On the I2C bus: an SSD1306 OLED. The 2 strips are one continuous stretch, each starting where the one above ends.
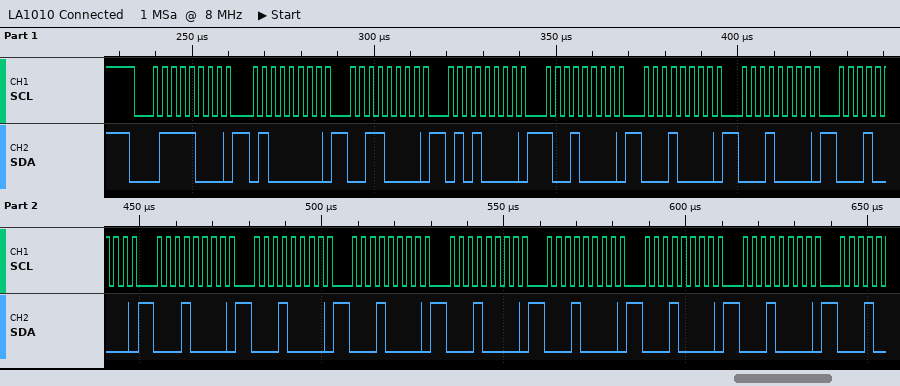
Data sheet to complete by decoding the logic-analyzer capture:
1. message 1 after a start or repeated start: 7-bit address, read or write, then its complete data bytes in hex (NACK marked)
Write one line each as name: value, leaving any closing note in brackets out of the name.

message 1 after a start or repeated start: 7-bit address, read or write, then its complete data bytes in hex: 0x3C write: 40 30 50 90 10 10 10 10 10 10 10 10 10 10
